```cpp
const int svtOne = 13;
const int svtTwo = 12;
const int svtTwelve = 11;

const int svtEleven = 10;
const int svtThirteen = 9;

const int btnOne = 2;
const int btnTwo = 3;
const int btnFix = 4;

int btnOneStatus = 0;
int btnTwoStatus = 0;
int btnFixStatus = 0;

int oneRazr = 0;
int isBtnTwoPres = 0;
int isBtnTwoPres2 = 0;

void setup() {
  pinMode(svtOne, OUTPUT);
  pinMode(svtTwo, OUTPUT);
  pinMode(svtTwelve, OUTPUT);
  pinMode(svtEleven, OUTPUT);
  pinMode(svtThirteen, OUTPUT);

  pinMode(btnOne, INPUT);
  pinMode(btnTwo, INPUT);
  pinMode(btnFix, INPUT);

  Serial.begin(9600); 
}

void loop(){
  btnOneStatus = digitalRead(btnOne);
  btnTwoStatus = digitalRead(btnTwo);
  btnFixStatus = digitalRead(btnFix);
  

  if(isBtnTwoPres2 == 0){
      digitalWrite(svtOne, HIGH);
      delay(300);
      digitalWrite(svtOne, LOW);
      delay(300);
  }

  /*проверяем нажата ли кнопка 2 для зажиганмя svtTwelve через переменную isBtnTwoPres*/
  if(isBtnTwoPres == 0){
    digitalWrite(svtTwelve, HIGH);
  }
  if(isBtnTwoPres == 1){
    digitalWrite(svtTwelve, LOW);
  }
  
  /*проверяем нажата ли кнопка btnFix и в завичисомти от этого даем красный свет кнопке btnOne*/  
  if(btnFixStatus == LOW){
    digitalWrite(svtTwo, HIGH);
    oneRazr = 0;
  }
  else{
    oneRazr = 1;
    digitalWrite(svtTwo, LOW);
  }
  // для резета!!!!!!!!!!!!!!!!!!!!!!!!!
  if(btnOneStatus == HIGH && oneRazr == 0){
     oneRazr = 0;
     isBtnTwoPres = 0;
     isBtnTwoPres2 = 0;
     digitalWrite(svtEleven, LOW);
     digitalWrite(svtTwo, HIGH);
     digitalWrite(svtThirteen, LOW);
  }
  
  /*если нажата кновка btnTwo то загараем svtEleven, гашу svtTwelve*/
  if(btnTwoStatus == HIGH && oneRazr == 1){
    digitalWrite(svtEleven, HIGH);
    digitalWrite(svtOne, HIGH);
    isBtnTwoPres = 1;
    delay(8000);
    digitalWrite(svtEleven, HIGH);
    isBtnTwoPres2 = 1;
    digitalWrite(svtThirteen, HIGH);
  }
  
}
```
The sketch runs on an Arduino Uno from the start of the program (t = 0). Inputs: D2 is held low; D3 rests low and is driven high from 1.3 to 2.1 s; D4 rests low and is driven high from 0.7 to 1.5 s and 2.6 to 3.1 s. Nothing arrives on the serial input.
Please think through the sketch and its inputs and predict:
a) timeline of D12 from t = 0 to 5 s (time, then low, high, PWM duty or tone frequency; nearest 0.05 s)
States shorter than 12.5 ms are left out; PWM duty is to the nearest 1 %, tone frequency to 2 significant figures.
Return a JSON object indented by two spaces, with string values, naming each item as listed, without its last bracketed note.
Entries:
{
  "timeline of D12 from t = 0 to 5 s": "0 s low; 0.6 s high; 1.8 s low; 2.4 s high; 3.6 s low; 4.2 s high"
}
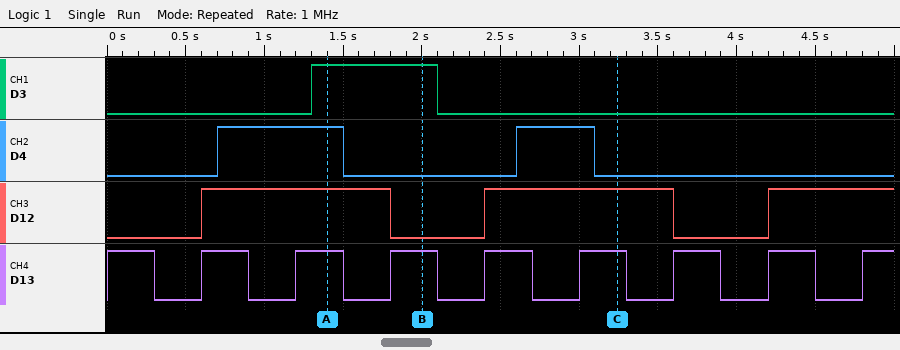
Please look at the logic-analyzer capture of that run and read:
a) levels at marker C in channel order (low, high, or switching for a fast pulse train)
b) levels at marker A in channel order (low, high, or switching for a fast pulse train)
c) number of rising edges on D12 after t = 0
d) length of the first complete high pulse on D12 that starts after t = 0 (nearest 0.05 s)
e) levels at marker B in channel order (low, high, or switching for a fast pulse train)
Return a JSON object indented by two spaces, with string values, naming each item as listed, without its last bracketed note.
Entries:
{
  "levels at marker C in channel order": "D3 low, D4 low, D12 high, D13 high",
  "levels at marker A in channel order": "D3 high, D4 high, D12 high, D13 high",
  "number of rising edges on D12 after t = 0": "3",
  "length of the first complete high pulse on D12 that starts after t = 0": "1.20 s",
  "levels at marker B in channel order": "D3 high, D4 low, D12 low, D13 high"
}
